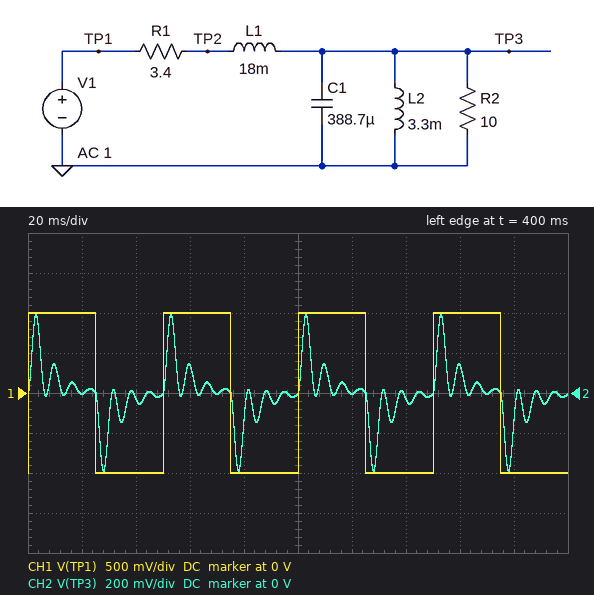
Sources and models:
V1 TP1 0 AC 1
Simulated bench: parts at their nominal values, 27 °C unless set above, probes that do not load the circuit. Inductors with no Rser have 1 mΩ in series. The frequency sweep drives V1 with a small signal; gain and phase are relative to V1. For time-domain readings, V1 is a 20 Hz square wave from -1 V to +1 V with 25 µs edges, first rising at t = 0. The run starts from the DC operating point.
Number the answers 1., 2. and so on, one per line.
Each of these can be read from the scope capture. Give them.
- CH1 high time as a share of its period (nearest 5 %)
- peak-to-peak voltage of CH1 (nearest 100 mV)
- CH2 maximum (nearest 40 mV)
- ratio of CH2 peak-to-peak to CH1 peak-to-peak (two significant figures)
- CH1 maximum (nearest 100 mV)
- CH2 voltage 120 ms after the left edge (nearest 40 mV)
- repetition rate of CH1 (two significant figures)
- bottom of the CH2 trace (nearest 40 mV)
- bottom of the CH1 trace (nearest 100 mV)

1. 50 %
2. 2.0 V
3. 400 mV
4. 0.39
5. 1.0 V
6. 0 V
7. 20 Hz
8. -400 mV
9. -1.0 V
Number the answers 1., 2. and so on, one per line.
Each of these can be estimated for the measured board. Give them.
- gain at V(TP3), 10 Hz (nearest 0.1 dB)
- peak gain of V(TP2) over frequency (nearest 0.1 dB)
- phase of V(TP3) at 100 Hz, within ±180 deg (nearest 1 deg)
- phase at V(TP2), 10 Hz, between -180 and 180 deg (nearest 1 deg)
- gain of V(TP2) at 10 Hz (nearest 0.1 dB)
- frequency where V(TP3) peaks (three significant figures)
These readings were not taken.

1. -24.9 dB
2. 0 dB
3. -5 deg
4. 68 deg
5. -8.7 dB
6. 150 Hz
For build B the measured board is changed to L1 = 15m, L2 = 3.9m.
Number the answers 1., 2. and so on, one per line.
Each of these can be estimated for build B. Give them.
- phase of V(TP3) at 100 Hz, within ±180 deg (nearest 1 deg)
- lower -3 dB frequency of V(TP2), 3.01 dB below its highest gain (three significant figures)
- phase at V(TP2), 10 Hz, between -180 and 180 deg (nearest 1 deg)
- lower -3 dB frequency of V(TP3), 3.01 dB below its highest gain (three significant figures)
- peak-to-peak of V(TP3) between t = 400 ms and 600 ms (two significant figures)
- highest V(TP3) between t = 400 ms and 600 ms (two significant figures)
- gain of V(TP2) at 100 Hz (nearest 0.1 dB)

1. -8 deg
2. 28.8 Hz
3. 70 deg
4. 115 Hz
5. 990 mV
6. 500 mV
7. -0.6 dB
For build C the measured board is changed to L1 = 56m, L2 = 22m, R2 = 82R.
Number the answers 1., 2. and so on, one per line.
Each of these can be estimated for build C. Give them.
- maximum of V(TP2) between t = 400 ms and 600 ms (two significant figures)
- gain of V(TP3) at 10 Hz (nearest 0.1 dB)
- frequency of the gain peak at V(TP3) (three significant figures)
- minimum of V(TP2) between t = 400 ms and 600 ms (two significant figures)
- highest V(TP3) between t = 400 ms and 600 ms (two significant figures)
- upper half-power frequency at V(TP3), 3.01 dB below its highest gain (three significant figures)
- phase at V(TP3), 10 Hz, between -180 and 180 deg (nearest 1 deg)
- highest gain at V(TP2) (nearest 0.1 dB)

1. 1.4 V
2. -12.5 dB
3. 64.0 Hz
4. -1.4 V
5. 1.1 V
6. 67.7 Hz
7. 34 deg
8. 0 dB
